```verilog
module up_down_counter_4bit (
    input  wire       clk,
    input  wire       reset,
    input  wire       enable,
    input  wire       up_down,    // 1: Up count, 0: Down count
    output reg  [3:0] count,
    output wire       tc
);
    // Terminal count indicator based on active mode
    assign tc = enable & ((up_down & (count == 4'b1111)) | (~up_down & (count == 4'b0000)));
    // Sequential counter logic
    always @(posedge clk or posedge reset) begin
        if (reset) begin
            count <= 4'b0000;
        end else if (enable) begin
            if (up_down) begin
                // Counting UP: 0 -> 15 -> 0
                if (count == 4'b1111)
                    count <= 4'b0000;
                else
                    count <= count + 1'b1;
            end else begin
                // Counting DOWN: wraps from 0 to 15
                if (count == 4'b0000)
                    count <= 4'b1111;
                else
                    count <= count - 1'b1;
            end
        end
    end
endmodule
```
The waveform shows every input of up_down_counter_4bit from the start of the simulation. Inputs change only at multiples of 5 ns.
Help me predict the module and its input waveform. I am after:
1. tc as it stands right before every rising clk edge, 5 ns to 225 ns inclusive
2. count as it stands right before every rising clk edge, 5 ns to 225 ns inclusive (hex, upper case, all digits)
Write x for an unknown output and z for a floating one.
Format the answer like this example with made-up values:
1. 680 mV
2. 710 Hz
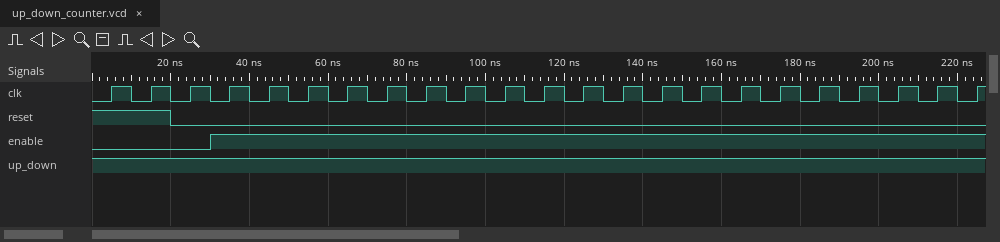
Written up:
1. 0 0 0 0 0 0 0 0 0 0 0 0 0 0 0 0 0 0 1 0 0 0 0
2. 0, 0, 0, 0, 1, 2, 3, 4, 5, 6, 7, 8, 9, A, B, C, D, E, F, 0, 1, 2, 3
